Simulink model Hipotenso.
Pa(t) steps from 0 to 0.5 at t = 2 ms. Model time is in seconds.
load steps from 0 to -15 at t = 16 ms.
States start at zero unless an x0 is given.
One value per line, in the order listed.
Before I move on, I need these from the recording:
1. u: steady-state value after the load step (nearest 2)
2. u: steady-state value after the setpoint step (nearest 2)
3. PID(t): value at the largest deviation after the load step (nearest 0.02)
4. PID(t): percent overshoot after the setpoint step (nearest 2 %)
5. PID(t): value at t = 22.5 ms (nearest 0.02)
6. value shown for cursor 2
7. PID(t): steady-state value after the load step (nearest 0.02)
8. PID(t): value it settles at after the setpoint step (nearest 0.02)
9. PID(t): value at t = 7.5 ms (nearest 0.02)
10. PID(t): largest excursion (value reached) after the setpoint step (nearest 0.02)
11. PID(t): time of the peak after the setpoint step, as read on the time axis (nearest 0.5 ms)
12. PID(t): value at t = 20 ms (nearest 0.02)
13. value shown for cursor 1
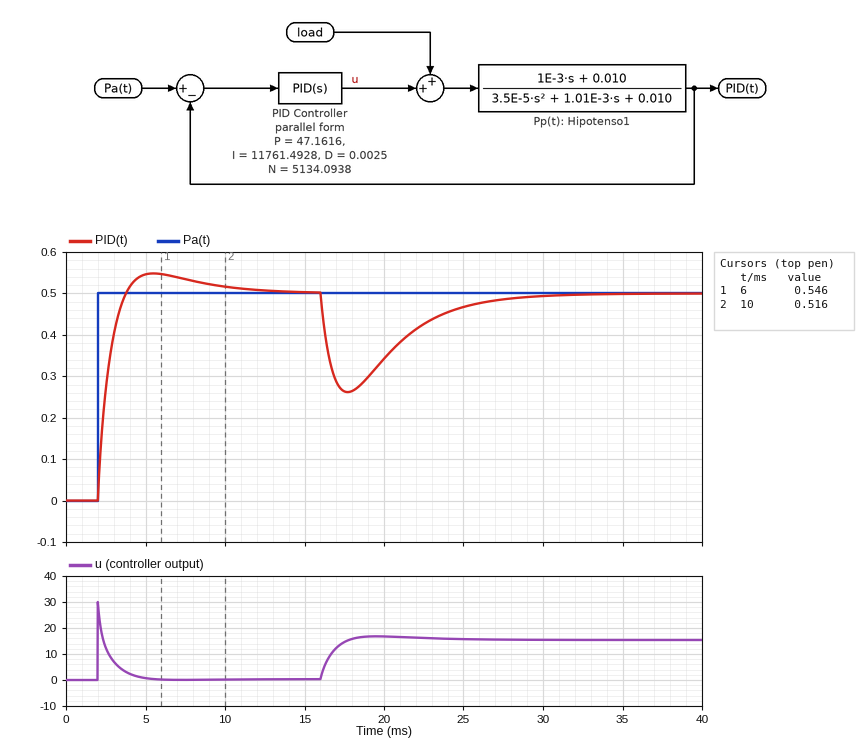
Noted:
16
0
0.26
10 %
0.42
0.516
0.50
0.50
0.54
0.54
5.5 ms
0.34
0.546
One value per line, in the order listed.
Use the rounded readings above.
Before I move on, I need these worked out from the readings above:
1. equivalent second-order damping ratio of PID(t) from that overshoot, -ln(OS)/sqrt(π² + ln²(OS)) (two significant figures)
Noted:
0.59
